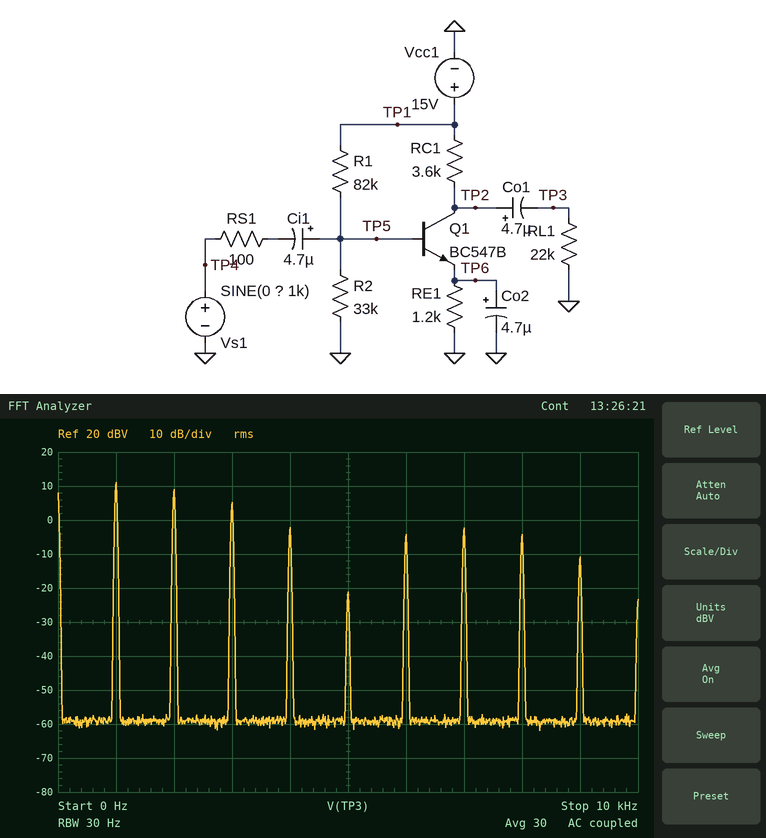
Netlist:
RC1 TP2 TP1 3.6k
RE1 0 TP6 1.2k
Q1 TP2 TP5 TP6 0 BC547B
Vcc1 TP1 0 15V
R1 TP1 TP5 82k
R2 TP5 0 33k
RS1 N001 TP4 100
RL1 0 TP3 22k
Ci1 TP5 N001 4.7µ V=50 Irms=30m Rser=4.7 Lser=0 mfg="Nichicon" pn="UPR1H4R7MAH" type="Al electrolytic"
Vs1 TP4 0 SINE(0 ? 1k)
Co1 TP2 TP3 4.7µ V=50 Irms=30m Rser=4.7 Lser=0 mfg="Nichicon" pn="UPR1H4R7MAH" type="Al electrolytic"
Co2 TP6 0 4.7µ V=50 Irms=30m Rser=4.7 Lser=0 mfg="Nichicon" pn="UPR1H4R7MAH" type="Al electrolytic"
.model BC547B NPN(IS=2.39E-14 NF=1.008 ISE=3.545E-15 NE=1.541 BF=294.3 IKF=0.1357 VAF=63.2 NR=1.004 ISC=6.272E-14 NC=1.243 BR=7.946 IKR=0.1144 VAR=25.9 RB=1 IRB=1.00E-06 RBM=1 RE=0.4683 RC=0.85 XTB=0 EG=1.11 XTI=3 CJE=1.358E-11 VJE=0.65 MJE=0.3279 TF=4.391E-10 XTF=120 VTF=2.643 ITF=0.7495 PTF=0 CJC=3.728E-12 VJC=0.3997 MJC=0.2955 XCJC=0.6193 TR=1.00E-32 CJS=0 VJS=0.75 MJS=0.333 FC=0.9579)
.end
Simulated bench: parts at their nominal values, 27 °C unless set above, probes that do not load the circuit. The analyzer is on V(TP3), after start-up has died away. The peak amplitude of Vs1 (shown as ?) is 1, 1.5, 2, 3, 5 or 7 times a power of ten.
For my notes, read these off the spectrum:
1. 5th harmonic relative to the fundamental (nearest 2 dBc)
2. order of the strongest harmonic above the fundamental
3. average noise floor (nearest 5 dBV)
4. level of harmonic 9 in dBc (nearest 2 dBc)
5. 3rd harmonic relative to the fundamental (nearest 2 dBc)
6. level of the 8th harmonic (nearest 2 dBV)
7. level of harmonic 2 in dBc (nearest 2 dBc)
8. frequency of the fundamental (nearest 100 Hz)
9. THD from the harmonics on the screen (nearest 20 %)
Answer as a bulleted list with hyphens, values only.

- -32 dBc
- 2
- -60 dBV
- -22 dBc
- -6 dBc
- -4 dBV
- -2 dBc
- 1.0 kHz
- 100 %
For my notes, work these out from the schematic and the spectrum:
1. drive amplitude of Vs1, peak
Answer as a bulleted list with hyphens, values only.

- 1 V
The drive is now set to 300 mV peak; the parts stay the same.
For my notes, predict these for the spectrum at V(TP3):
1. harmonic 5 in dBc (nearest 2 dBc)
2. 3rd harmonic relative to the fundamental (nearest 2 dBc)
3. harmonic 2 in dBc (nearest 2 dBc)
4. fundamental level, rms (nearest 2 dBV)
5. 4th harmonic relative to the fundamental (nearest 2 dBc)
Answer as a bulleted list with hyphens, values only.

- -14 dBc
- -22 dBc
- -6 dBc
- 14 dBV
- -16 dBc
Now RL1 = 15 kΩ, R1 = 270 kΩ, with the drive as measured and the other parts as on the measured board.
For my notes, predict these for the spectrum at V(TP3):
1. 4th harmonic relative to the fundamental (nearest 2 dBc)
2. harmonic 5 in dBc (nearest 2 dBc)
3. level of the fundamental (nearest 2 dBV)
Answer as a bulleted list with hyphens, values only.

- -6 dBc
- -10 dBc
- 8 dBV
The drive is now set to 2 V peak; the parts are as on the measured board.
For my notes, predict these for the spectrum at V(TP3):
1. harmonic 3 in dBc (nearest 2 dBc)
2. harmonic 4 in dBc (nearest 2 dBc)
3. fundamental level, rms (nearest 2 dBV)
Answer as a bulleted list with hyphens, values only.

- -4 dBc
- -8 dBc
- 10 dBV
